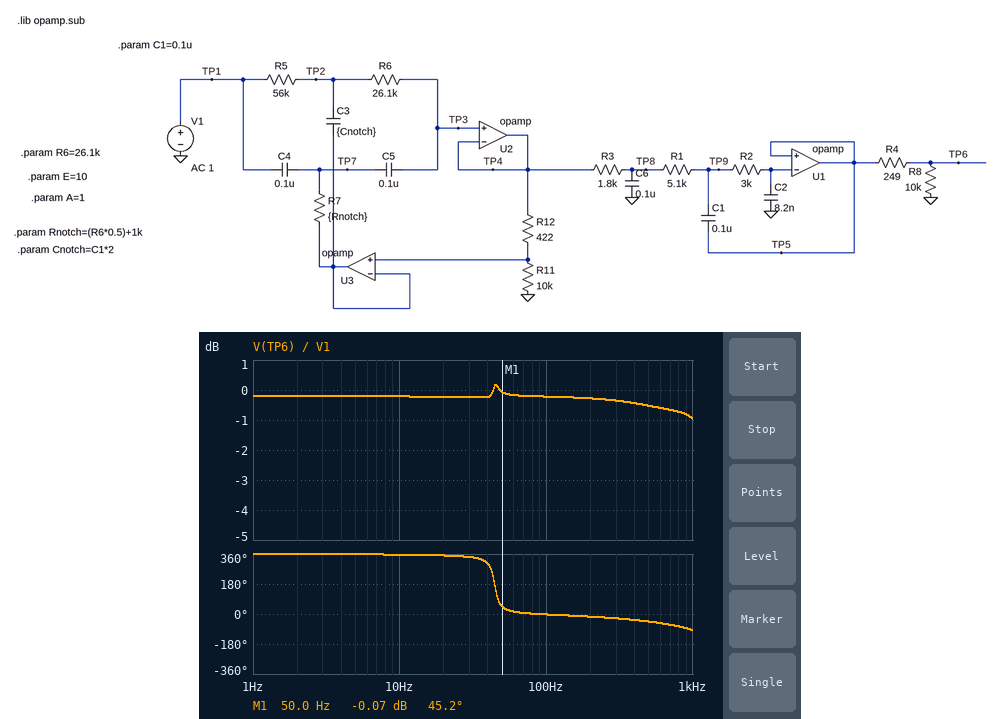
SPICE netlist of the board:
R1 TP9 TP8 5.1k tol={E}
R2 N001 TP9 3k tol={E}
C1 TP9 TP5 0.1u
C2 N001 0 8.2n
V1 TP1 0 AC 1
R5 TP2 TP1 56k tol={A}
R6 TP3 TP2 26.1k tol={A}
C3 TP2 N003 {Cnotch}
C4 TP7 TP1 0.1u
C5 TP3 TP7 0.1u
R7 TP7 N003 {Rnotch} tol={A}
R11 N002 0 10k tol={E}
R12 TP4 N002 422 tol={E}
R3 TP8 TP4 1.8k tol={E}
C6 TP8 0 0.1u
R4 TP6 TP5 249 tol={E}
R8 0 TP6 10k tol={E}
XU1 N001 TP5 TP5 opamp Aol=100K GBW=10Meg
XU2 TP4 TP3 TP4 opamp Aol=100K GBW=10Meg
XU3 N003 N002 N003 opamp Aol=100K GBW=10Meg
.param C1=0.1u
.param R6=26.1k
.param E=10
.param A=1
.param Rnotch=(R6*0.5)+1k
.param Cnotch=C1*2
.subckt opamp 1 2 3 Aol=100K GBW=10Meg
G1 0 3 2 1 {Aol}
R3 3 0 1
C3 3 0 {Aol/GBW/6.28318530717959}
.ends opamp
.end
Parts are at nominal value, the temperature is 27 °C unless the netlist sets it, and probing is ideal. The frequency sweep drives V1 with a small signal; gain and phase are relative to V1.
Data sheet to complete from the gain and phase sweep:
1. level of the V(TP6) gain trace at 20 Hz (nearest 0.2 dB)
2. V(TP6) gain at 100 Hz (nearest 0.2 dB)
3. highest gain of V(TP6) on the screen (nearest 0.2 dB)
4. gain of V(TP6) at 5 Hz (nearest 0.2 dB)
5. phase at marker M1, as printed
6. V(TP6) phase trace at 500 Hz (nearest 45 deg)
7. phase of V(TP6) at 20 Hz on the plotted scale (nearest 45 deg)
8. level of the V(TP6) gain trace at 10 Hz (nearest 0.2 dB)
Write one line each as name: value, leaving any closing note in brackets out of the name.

level of the V(TP6) gain trace at 20 Hz: -0.2 dB
V(TP6) gain at 100 Hz: -0.2 dB
highest gain of V(TP6) on the screen: 0.2 dB
gain of V(TP6) at 5 Hz: -0.2 dB
phase at marker M1, as printed: 45.2 deg
V(TP6) phase trace at 500 Hz: -45 deg
phase of V(TP6) at 20 Hz on the plotted scale: 360 deg
level of the V(TP6) gain trace at 10 Hz: -0.2 dB
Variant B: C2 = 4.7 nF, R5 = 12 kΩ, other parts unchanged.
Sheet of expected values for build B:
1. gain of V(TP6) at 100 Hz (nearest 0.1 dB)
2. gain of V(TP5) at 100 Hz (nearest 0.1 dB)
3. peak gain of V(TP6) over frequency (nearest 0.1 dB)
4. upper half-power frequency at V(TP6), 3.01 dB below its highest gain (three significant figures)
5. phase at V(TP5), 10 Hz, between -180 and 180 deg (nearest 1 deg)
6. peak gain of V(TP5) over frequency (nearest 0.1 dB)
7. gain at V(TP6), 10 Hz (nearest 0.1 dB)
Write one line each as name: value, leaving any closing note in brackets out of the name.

gain of V(TP6) at 100 Hz: -1.3 dB
gain of V(TP5) at 100 Hz: -1.1 dB
peak gain of V(TP6) over frequency: -0.2 dB
upper half-power frequency at V(TP6), 3.01 dB below its highest gain: 1.88 kHz
phase at V(TP5), 10 Hz, between -180 and 180 deg: -2 deg
peak gain of V(TP5) over frequency: 0 dB
gain at V(TP6), 10 Hz: -0.2 dB
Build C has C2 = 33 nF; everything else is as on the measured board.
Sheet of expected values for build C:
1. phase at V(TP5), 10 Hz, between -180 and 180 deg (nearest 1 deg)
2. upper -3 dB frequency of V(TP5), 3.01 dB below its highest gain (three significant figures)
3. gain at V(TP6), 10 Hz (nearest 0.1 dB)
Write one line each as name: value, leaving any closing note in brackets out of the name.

phase at V(TP5), 10 Hz, between -180 and 180 deg: -5 deg
upper -3 dB frequency of V(TP5), 3.01 dB below its highest gain: 517 Hz
gain at V(TP6), 10 Hz: -0.2 dB
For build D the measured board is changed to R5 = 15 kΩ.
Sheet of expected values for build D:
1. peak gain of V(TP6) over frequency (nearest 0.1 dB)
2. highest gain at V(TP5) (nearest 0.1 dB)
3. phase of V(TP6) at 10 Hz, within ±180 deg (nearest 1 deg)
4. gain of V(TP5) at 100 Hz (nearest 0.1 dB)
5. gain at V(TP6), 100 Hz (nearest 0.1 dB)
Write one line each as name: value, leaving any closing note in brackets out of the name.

peak gain of V(TP6) over frequency: -0.2 dB
highest gain at V(TP5): 0 dB
phase of V(TP6) at 10 Hz, within ±180 deg: -2 deg
gain of V(TP5) at 100 Hz: -0.7 dB
gain at V(TP6), 100 Hz: -0.9 dB
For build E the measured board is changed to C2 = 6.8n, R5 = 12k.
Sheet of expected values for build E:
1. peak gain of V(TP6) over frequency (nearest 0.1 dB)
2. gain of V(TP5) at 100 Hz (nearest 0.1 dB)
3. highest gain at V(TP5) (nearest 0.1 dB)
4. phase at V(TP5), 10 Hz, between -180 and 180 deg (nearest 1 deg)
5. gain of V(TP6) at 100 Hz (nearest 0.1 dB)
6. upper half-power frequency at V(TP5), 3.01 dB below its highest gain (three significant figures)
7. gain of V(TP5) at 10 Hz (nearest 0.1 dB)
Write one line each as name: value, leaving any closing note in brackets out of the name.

peak gain of V(TP6) over frequency: -0.2 dB
gain of V(TP5) at 100 Hz: -1.1 dB
highest gain at V(TP5): 0 dB
phase at V(TP5), 10 Hz, between -180 and 180 deg: -2 deg
gain of V(TP6) at 100 Hz: -1.3 dB
upper half-power frequency at V(TP5), 3.01 dB below its highest gain: 1.53 kHz
gain of V(TP5) at 10 Hz: 0 dB
